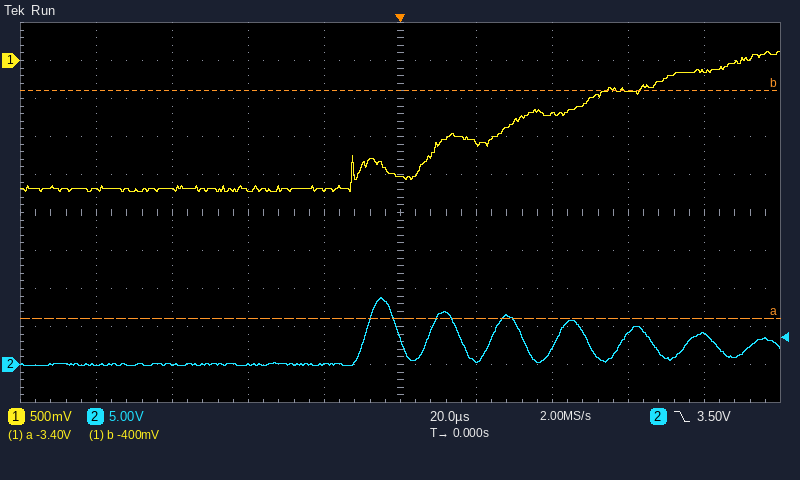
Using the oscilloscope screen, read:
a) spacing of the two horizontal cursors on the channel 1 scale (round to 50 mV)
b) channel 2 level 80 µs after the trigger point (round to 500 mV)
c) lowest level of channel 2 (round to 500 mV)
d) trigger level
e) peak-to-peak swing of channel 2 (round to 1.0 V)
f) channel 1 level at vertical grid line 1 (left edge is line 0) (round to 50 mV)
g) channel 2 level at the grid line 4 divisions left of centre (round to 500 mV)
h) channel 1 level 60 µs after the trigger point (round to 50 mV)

3.00 V
4.0 V
0.0 V
3.50 V
9.0 V
-1.70 V
0.0 V
-400 mV
